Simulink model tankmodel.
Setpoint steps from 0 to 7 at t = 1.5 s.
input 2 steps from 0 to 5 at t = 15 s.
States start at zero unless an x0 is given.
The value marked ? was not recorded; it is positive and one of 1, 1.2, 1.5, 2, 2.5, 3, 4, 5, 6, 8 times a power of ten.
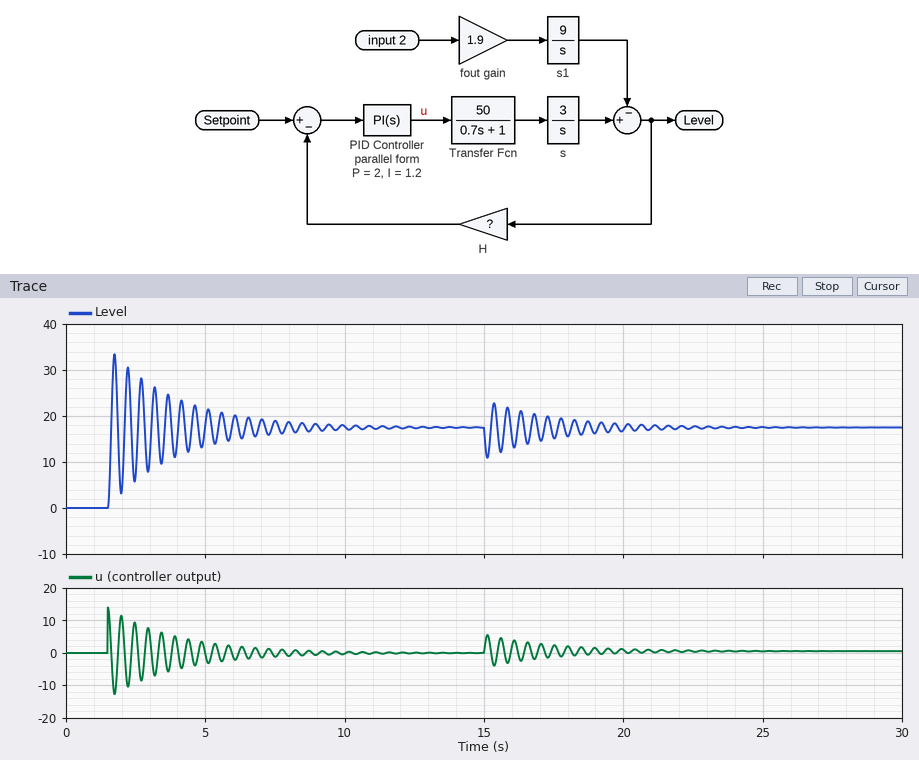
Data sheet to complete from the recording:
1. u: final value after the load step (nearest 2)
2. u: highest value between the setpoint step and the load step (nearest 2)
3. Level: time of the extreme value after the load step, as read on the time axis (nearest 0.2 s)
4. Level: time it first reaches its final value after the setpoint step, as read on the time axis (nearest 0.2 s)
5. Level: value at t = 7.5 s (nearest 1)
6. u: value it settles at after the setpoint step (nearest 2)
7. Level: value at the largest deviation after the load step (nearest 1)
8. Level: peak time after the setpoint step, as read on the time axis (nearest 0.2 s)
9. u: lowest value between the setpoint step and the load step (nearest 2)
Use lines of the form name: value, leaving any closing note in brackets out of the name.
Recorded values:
u: final value after the load step: 0
u: highest value between the setpoint step and the load step: 14
Level: time of the extreme value after the load step, as read on the time axis: 15.2 s
Level: time it first reaches its final value after the setpoint step, as read on the time axis: 1.6 s
Level: value at t = 7.5 s: 19
u: value it settles at after the setpoint step: 0
Level: value at the largest deviation after the load step: 11
Level: peak time after the setpoint step, as read on the time axis: 1.8 s
u: lowest value between the setpoint step and the load step: -12
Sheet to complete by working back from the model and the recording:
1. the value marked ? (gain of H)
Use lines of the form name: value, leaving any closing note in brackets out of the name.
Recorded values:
the value marked ?: 0.4
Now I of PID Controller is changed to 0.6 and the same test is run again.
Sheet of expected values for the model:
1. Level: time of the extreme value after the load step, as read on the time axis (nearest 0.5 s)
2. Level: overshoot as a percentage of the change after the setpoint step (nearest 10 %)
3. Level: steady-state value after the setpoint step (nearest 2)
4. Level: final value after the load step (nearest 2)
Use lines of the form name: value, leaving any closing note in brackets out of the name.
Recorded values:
Level: time of the extreme value after the load step, as read on the time axis: 15.0 s
Level: overshoot as a percentage of the change after the setpoint step: 90 %
Level: steady-state value after the setpoint step: 18
Level: final value after the load step: 18
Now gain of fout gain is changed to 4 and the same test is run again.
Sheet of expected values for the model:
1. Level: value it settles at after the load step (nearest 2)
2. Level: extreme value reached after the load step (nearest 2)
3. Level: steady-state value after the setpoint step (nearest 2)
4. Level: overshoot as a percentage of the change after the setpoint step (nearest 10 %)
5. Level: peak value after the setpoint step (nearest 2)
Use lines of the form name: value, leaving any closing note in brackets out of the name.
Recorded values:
Level: value it settles at after the load step: 18
Level: extreme value reached after the load step: 4
Level: steady-state value after the setpoint step: 18
Level: overshoot as a percentage of the change after the setpoint step: 90 %
Level: peak value after the setpoint step: 34
